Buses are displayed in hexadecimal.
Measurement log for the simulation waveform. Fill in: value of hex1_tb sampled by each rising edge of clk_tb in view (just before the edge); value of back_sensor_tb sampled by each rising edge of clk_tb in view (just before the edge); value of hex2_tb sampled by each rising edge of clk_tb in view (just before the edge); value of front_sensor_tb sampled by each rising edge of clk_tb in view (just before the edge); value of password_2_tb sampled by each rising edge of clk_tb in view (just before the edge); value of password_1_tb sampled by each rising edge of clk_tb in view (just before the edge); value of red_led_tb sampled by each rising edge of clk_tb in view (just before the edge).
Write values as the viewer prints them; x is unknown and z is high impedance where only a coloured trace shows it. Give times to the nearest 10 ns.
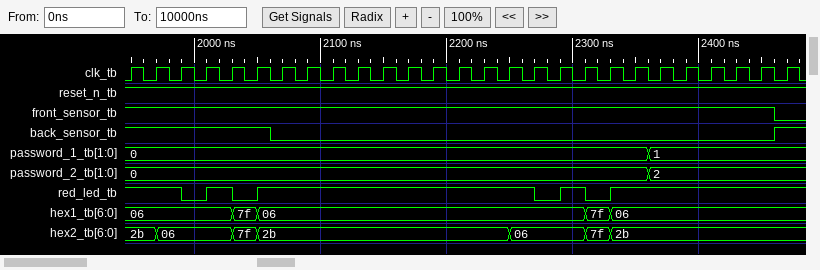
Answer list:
06, 06, 06, 06, 06, 7f, 06, 06, 06, 06, 06, 06, 06, 06, 06, 06, 06, 06, 06, 7f, 06, 06, 06, 06, 06, 06, 06
1 1 1 1 1 1 0 0 0 0 0 0 0 0 0 0 0 0 0 0 0 0 0 0 0 0 1
2b, 2b, 06, 06, 06, 7f, 2b, 2b, 2b, 2b, 2b, 2b, 2b, 2b, 2b, 2b, 06, 06, 06, 7f, 2b, 2b, 2b, 2b, 2b, 2b, 2b
1 1 1 1 1 1 1 1 1 1 1 1 1 1 1 1 1 1 1 1 1 1 1 1 1 1 0
0, 0, 0, 0, 0, 0, 0, 0, 0, 0, 0, 0, 0, 0, 0, 0, 0, 0, 0, 0, 0, 2, 2, 2, 2, 2, 2
0, 0, 0, 0, 0, 0, 0, 0, 0, 0, 0, 0, 0, 0, 0, 0, 0, 0, 0, 0, 0, 1, 1, 1, 1, 1, 1
1 1 1 0 1 0 1 1 1 1 1 1 1 1 1 1 1 0 1 0 1 1 1 1 1 1 1
